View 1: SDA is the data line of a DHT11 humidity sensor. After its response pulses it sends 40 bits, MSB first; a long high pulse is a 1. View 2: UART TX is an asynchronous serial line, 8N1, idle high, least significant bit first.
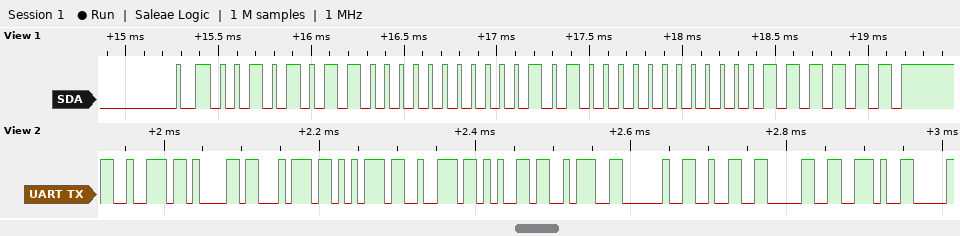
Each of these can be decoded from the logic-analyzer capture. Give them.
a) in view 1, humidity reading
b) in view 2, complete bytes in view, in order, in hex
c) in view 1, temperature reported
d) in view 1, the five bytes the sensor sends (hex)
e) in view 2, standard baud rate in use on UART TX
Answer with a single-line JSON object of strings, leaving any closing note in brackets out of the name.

{"in view 1, humidity reading": "43 %", "in view 2, complete bytes in view, in order, in hex": "72 61 74 75 72 65 3A 20 32 30 2E", "in view 1, temperature reported": "20.0 °C", "in view 1, the five bytes the sensor sends": "2B 00 14 00 3F", "in view 2, standard baud rate in use on UART TX": "115200 baud"}
